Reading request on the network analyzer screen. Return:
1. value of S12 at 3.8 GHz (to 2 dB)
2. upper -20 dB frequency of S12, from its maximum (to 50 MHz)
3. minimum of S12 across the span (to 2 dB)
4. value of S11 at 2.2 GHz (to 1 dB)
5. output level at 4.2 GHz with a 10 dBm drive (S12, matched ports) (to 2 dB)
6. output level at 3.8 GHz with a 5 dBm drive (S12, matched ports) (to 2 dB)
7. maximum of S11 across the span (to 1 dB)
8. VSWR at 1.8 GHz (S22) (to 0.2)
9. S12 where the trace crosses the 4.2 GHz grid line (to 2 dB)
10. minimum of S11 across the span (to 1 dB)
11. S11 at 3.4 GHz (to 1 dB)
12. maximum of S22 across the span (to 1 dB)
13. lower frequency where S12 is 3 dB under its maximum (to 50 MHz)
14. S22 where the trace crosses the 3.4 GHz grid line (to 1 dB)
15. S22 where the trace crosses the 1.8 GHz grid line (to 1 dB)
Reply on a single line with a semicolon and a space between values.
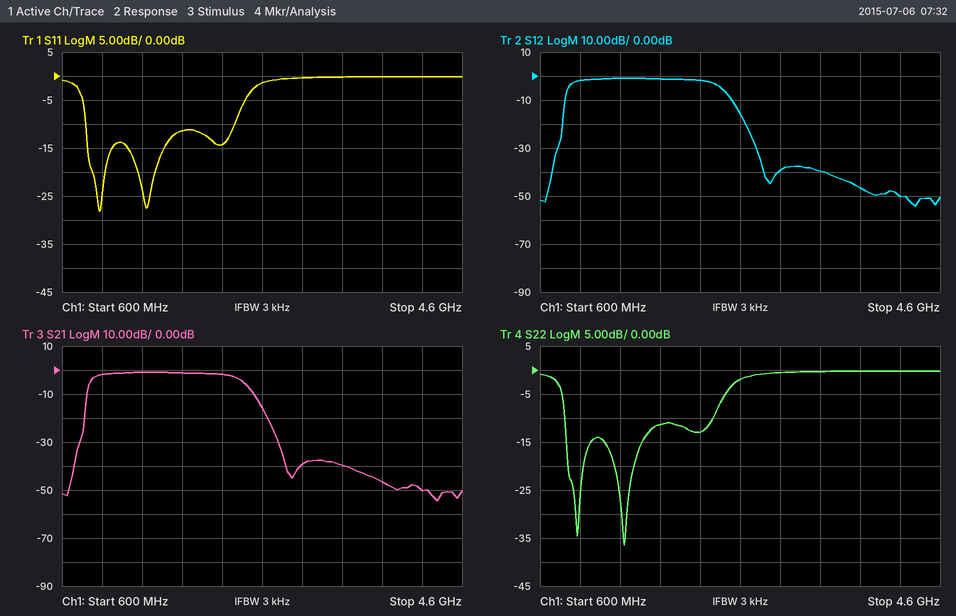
-46 dB; 2.65 GHz; -54 dB; -14 dB; -40 dBm; -42 dBm; 0 dB; 1.8; -50 dB; -28 dB; 0 dB; 0 dB; 900 MHz; 0 dB; -11 dB
